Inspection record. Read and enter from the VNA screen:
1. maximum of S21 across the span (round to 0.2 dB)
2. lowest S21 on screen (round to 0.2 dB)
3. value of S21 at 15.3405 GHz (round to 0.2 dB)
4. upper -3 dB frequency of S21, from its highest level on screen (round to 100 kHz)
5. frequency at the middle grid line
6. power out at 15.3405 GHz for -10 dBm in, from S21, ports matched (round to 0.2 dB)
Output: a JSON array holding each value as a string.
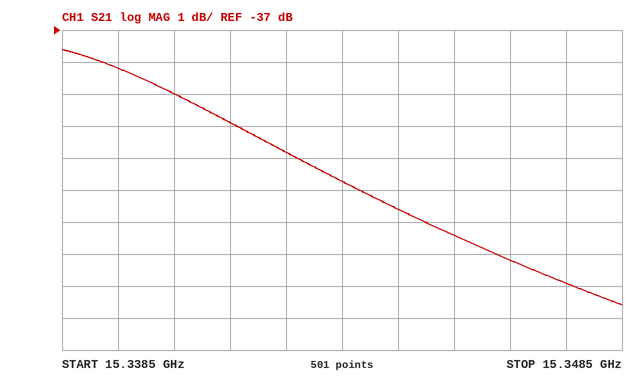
["-37.6 dB", "-45.6 dB", "-39.0 dB", "15.3423 GHz", "15.3435 GHz", "-49.0 dBm"]
